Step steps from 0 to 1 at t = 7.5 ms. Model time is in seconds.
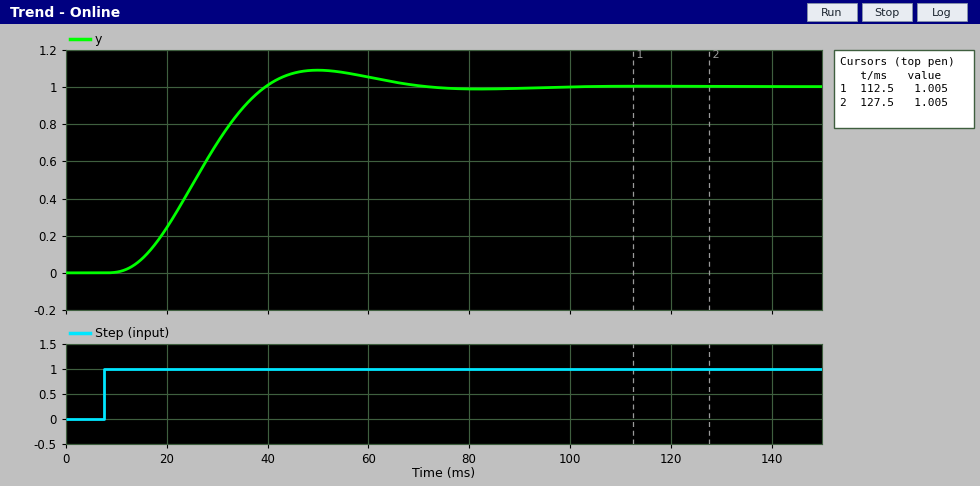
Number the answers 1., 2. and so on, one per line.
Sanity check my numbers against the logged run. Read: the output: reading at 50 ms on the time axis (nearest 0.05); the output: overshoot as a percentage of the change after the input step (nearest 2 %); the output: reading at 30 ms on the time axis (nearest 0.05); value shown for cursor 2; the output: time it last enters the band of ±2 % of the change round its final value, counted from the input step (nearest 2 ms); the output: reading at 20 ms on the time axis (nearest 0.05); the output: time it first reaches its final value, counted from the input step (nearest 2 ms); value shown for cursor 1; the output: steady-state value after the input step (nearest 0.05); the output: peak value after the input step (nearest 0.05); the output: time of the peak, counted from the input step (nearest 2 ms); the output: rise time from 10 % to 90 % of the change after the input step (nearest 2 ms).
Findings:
1. 1.10
2. 8 %
3. 0.70
4. 1.005
5. 58 ms
6. 0.25
7. 32 ms
8. 1.005
9. 1.00
10. 1.10
11. 42 ms
12. 20 ms
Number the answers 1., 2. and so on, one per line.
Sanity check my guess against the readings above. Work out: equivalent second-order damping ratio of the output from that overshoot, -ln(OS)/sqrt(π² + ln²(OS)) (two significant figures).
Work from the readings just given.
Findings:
1. 0.63
